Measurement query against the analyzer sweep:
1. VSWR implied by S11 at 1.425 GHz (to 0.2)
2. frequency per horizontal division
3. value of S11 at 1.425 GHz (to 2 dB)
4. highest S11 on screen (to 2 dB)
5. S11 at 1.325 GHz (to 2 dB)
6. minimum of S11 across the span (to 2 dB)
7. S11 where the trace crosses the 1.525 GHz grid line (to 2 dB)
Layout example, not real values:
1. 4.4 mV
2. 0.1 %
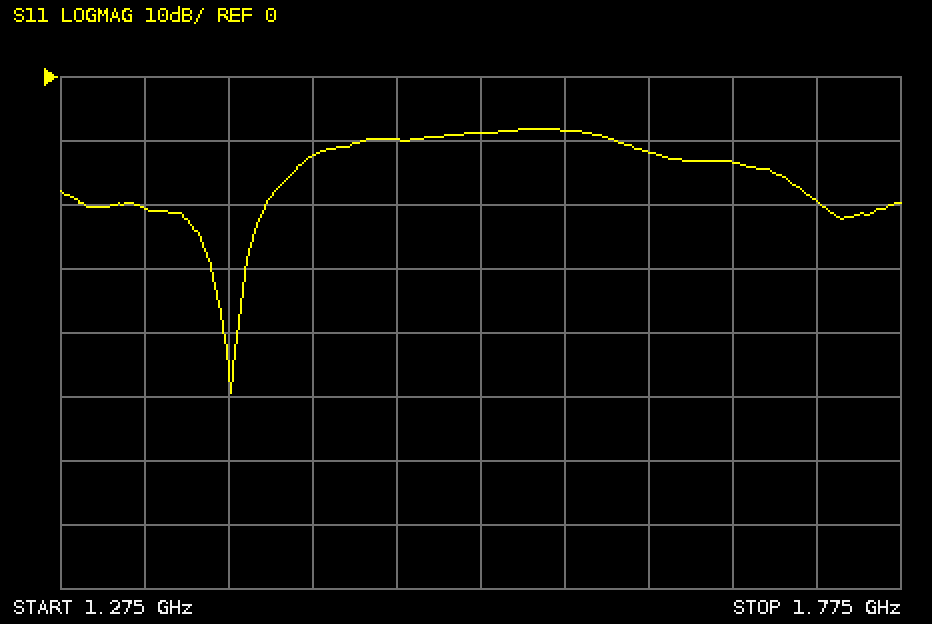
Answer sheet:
1. 1.6
2. 50 MHz
3. -12 dB
4. -8 dB
5. -20 dB
6. -50 dB
7. -8 dB
